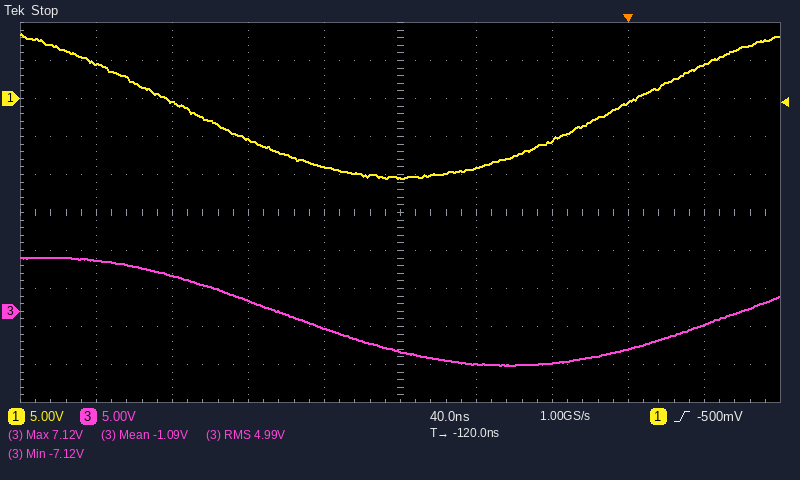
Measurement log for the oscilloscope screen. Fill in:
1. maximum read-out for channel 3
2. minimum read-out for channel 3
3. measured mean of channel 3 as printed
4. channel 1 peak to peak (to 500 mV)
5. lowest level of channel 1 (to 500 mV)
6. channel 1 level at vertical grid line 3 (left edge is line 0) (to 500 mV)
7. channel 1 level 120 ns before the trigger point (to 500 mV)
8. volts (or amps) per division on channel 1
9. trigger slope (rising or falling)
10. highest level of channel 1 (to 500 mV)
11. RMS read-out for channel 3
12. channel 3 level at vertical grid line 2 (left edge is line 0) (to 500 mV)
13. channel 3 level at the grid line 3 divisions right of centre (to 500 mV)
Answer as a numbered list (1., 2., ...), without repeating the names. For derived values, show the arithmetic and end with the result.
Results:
1. 7.12 V
2. -7.12 V
3. -1.09 V
4. 8.5 V − (-10.5 V) = 19.0 V
5. -10.5 V
6. -5.5 V
7. -10.5 V
8. 5 V
9. rising
10. 8.5 V
11. 4.99 V
12. 4.5 V
13. -5.0 V
